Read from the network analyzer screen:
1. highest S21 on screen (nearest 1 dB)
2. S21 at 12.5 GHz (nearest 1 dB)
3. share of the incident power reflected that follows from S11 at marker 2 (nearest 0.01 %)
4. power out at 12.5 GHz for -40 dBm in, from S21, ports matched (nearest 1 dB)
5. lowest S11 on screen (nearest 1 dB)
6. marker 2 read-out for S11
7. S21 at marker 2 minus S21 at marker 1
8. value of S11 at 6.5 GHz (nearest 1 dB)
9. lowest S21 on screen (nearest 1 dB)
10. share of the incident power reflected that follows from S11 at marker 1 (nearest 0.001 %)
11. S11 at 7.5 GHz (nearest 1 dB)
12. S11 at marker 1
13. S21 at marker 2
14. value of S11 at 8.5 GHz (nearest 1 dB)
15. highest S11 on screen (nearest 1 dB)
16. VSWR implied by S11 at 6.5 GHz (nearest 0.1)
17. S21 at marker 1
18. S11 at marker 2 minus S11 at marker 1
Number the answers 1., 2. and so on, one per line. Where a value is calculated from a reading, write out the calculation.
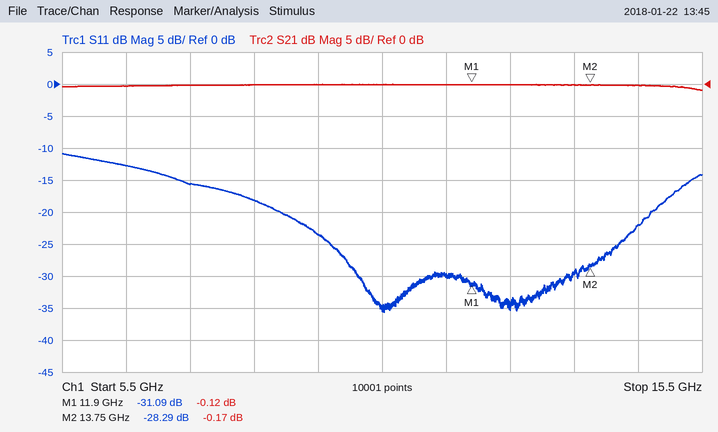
1. 0 dB
2. 0 dB
3. 10^(-28.29/10) ≈ 0.15 %
4. -40 dBm + (0 dB) = -40 dBm
5. -36 dB
6. -28.29 dB
7. -0.17 − (-0.12) = -0.05 dB
8. -13 dB
9. -1 dB
10. 10^(-31.09/10) ≈ 0.078 %
11. -16 dB
12. -31.09 dB
13. -0.17 dB
14. -18 dB
15. -11 dB
16. |Γ| = 10^(-13/20) = 0.2239; VSWR = (1 + 0.2239)/(1 − 0.2239) ≈ 1.6
17. -0.12 dB
18. -28.29 − (-31.09) = 2.80 dB
